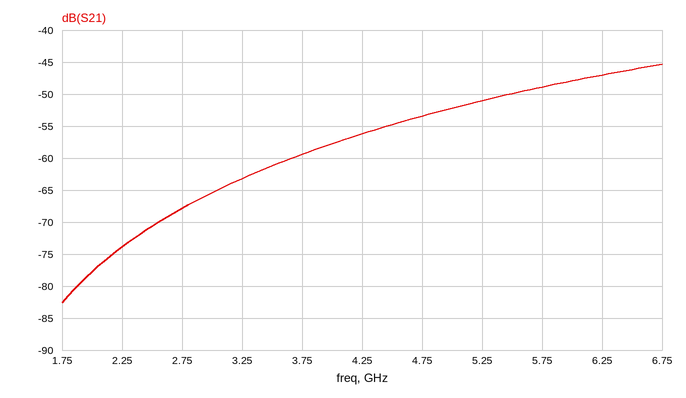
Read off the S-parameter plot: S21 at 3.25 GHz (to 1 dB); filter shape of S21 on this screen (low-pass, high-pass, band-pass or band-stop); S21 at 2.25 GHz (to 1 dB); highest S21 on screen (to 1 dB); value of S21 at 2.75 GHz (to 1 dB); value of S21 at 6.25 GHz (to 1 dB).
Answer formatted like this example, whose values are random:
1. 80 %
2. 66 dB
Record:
1. -63 dB
2. high-pass
3. -74 dB
4. -45 dB
5. -68 dB
6. -47 dB
